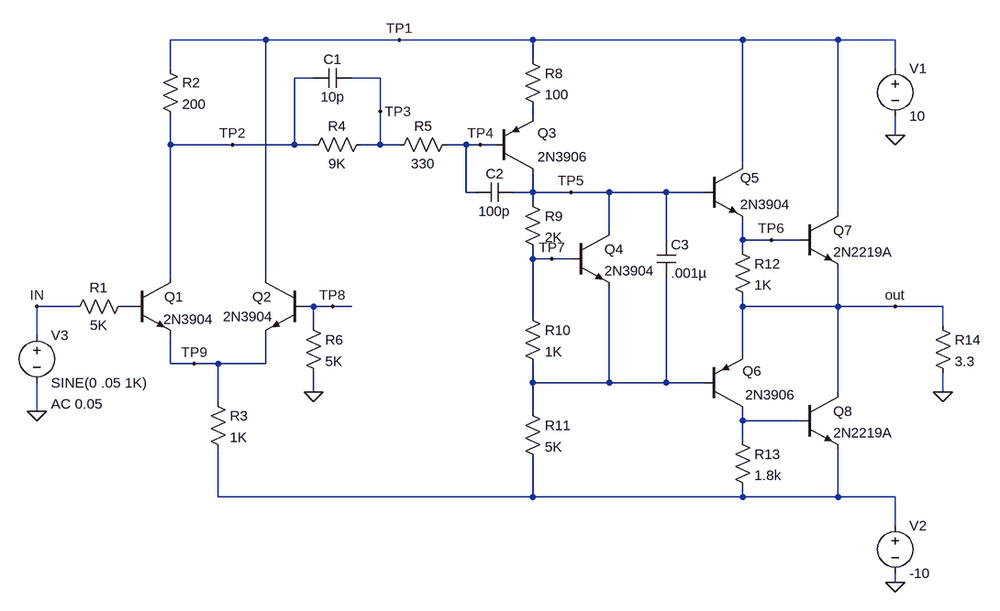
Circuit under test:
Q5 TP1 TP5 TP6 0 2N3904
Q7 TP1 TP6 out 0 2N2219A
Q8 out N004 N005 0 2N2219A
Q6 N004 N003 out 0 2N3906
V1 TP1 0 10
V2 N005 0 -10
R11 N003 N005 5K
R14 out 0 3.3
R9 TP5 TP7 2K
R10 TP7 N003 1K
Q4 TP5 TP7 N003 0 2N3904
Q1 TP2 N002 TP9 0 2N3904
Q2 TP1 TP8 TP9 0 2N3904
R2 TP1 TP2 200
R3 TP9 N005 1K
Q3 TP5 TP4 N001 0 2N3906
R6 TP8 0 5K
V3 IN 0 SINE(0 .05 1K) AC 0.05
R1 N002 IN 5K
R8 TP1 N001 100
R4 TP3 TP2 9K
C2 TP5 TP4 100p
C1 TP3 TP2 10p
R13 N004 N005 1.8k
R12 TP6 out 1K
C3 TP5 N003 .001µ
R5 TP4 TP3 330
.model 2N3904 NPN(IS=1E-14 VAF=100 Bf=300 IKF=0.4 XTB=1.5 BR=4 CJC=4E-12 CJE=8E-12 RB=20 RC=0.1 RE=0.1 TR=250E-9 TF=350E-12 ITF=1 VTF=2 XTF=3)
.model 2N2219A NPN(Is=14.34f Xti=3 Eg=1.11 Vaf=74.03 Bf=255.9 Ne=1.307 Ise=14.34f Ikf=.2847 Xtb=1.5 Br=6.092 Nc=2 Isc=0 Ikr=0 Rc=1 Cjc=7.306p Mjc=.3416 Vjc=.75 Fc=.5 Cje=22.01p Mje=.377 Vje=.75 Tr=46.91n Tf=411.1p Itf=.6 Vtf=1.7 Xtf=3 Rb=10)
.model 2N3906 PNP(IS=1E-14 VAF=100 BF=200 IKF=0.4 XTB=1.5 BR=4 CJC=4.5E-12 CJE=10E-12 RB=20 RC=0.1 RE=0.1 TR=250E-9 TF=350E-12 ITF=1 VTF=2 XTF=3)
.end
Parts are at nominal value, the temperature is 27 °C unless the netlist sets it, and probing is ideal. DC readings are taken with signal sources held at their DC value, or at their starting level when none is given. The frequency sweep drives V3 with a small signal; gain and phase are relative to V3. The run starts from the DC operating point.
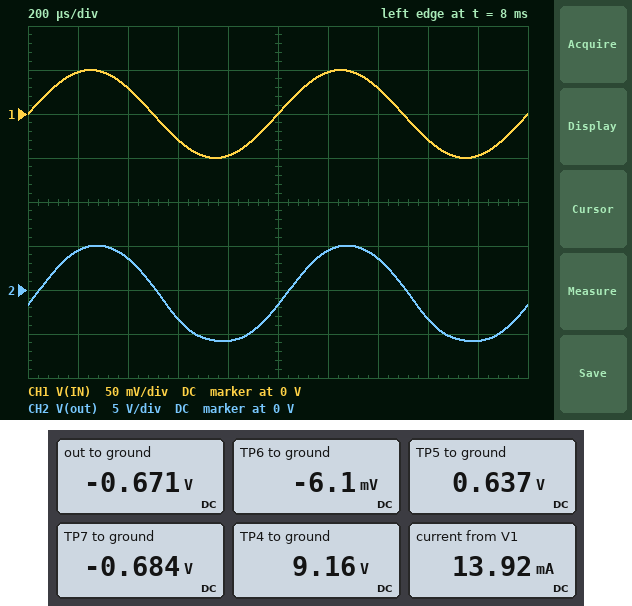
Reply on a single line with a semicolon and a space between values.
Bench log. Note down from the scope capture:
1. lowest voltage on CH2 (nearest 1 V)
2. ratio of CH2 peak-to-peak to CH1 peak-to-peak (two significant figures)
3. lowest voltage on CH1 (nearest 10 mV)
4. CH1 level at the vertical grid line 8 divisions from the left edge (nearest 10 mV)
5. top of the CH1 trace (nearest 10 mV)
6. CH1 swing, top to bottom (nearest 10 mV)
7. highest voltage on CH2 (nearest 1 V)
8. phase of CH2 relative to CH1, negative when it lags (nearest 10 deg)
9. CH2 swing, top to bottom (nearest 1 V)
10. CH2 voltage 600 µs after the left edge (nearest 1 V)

-6 V; 110; -50 mV; -30 mV; 50 mV; 100 mV; 5 V; -10 deg; 11 V; -3 V
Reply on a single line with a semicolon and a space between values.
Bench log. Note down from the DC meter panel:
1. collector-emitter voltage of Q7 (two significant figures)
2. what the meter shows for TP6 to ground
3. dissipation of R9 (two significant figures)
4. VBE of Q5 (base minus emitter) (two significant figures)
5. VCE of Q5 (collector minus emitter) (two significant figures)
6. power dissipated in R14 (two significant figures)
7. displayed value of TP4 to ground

11 V; -6.1 mV; 870 µW; 640 mV; 10 V; 140 mW; 9.16 V
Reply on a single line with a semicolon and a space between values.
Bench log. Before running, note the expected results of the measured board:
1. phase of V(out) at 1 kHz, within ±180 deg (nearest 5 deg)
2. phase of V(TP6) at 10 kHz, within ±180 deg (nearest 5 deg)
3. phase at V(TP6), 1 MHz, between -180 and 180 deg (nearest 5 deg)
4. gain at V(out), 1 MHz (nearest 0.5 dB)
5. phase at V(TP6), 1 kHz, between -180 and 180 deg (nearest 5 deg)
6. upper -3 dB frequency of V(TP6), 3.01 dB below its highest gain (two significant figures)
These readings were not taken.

-10 deg; -60 deg; -110 deg; -4.5 dB; -10 deg; 5.4 kHz
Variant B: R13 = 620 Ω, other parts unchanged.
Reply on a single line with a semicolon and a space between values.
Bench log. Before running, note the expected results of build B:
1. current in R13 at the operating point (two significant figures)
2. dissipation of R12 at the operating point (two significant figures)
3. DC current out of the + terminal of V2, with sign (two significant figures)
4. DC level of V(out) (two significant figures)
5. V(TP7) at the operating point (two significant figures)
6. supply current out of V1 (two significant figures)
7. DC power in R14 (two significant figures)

1.3 mA; 430 µW; -210 mA; -640 mV; -670 mV; 13 mA; 130 mW
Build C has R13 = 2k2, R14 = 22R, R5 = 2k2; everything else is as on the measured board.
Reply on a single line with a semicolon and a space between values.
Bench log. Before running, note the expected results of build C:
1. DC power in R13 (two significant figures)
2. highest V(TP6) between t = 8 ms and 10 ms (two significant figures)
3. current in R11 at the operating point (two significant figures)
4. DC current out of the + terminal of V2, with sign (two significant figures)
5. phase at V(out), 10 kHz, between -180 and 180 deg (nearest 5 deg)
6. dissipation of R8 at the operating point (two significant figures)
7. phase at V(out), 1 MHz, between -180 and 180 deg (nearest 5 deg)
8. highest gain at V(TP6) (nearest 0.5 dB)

260 µW; 6.1 V; 1.6 mA; -69 mA; -65 deg; 270 µW; -115 deg; 42.5 dB
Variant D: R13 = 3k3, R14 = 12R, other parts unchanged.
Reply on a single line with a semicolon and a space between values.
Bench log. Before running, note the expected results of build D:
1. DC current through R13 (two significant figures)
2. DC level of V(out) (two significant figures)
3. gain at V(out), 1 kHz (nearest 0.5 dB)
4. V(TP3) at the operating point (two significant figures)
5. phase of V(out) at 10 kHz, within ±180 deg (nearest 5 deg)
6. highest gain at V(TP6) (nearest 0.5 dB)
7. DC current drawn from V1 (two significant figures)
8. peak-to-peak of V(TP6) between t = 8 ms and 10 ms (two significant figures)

230 µA; -730 mV; 42.5 dB; 9.2 V; -65 deg; 43.0 dB; 18 mA; 14 V
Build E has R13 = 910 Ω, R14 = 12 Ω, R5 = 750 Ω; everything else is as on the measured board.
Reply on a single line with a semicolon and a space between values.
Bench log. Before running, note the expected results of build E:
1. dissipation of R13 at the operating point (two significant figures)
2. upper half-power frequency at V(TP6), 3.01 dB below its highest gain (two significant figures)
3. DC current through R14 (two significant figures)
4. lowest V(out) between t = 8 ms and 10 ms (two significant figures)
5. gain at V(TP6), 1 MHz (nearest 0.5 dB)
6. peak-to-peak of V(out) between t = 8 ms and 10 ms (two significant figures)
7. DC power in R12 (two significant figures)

640 µW; 5.0 kHz; 66 mA; -7.0 V; -4.5 dB; 13 V; 450 µW
